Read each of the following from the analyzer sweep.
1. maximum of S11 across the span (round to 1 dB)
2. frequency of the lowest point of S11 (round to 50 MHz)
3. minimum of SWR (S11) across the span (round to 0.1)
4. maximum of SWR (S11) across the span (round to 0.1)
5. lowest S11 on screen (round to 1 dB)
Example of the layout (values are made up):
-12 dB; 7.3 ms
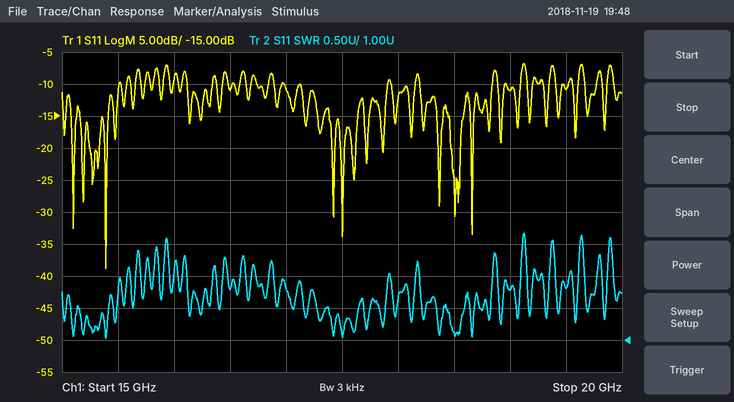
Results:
-7 dB; 15.40 GHz; 1.0; 2.7; -39 dB
